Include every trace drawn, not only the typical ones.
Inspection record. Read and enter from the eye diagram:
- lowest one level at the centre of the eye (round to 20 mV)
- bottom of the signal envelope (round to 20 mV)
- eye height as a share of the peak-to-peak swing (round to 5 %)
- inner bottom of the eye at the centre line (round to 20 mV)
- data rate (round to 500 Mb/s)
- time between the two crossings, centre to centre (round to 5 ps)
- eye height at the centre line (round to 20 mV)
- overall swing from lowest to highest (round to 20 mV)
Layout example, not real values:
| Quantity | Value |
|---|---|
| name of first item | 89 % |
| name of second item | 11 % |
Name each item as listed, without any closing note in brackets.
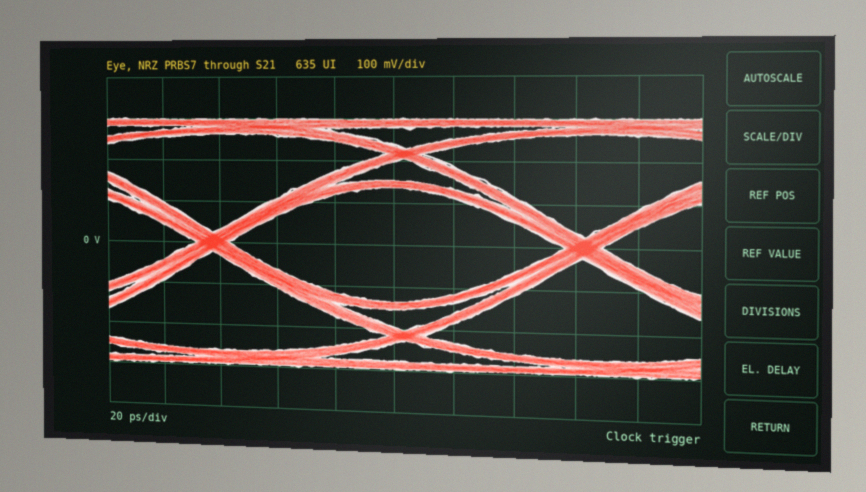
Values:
| Quantity | Value |
|---|---|
| lowest one level at the centre of the eye | 140 mV |
| bottom of the signal envelope | -300 mV |
| eye height as a share of the peak-to-peak swing | 45 % |
| inner bottom of the eye at the centre line | -140 mV |
| data rate | 8.0 Gb/s |
| time between the two crossings, centre to centre | 125 ps |
| eye height at the centre line | 280 mV |
| overall swing from lowest to highest | 600 mV |
